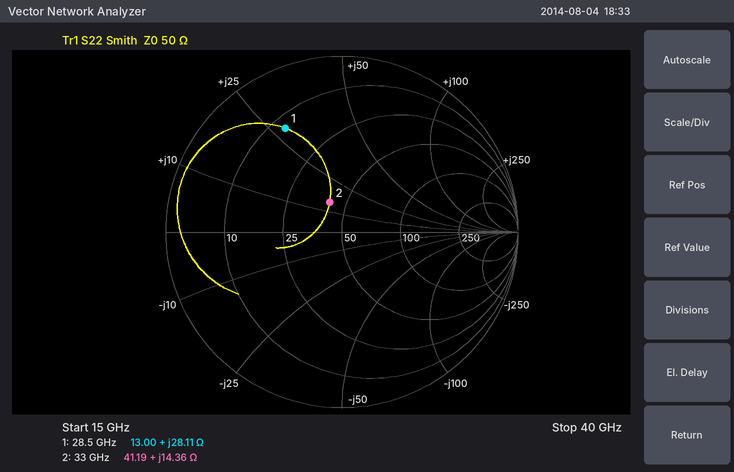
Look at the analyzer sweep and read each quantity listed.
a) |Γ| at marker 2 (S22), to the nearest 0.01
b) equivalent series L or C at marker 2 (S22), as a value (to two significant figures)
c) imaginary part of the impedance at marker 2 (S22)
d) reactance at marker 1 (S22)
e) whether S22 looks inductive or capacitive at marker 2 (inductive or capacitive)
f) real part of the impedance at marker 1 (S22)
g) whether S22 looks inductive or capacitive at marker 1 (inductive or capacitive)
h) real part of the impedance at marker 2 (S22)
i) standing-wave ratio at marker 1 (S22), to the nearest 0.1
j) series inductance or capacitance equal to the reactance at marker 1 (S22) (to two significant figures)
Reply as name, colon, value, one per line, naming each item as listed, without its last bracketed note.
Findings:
|Γ| at marker 2 (S22), to the nearest 0.01: 0.18
equivalent series L or C at marker 2 (S22), as a value: 69 pH
imaginary part of the impedance at marker 2: +14.36 Ω
reactance at marker 1: +28.11 Ω
whether S22 looks inductive or capacitive at marker 2: inductive
real part of the impedance at marker 1: 13.00 Ω
whether S22 looks inductive or capacitive at marker 1: inductive
real part of the impedance at marker 2: 41.19 Ω
standing-wave ratio at marker 1 (S22), to the nearest 0.1: 5.1
series inductance or capacitance equal to the reactance at marker 1 (S22): 160 pH
